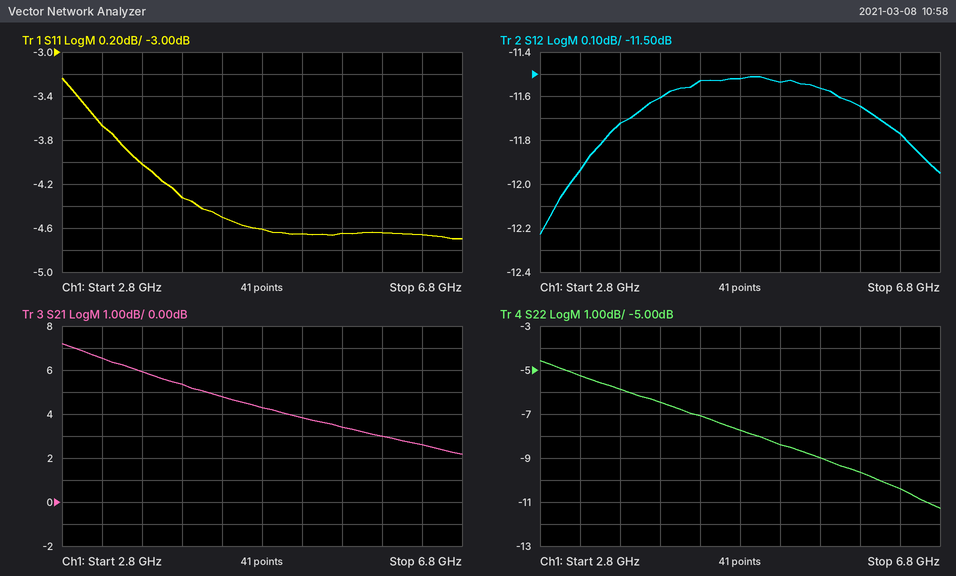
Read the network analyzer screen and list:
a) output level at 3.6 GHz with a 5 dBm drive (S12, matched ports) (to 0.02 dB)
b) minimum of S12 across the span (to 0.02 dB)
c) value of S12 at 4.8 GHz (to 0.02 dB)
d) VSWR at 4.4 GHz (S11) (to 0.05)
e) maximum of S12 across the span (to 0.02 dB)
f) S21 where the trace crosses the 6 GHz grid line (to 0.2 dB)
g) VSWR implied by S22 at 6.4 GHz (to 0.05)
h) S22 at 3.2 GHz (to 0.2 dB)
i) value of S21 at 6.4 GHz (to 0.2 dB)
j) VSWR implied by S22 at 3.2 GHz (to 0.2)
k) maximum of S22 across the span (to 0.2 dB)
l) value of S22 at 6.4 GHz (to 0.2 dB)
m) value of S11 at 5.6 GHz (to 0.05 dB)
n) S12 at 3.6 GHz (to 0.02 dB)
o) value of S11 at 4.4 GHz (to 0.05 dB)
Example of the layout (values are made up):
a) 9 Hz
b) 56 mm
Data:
a) -6.72 dBm
b) -12.22 dB
c) -11.52 dB
d) 3.95
e) -11.52 dB
f) 3.0 dB
g) 1.85
h) -5.2 dB
i) 2.6 dB
j) 3.4
k) -4.6 dB
l) -10.4 dB
m) -4.65 dB
n) -11.72 dB
o) -4.50 dB
